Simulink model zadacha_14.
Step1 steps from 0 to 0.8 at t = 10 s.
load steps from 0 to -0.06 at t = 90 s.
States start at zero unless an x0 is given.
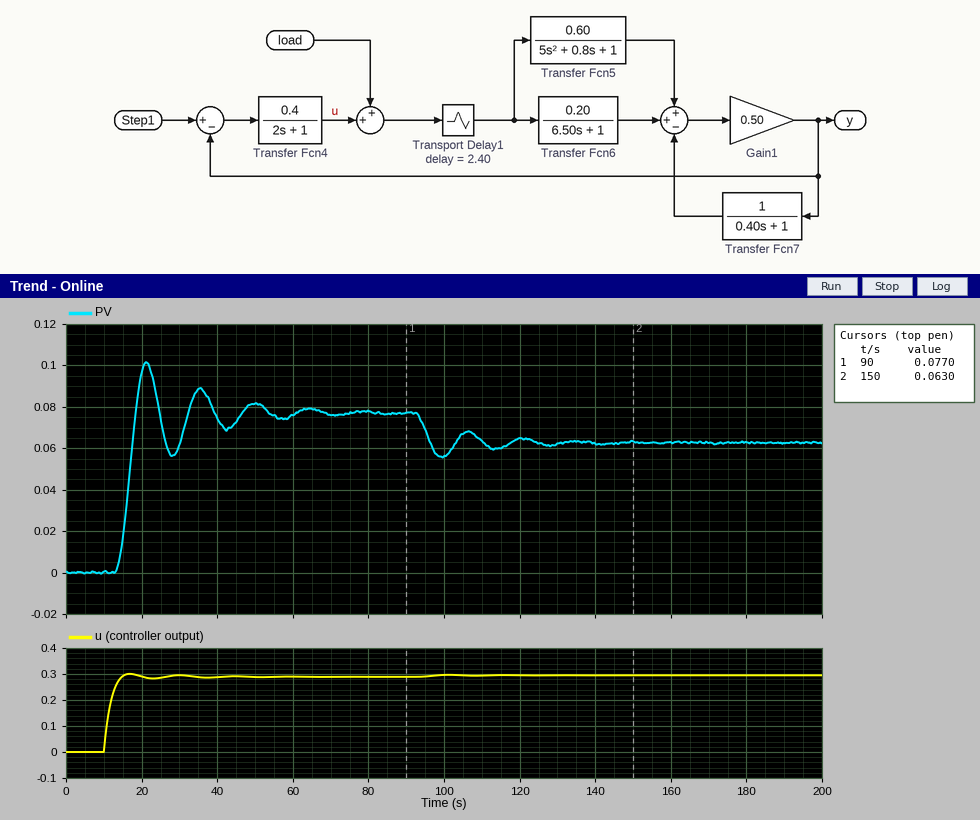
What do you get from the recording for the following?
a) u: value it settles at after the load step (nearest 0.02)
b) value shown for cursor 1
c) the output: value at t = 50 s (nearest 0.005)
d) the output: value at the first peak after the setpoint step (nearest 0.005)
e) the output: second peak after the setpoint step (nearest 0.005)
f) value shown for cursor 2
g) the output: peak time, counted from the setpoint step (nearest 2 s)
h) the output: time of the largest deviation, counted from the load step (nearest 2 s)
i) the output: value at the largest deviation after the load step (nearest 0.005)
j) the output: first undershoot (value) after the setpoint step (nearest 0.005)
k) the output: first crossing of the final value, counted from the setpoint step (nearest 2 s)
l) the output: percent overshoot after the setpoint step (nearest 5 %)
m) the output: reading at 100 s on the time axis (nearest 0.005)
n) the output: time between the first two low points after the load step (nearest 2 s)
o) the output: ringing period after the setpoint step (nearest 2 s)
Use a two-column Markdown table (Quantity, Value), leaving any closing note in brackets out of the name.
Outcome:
| Quantity | Value |
|---|---|
| u: value it settles at after the load step | 0.30 |
| value shown for cursor 1 | 0.0770 |
| the output: value at t = 50 s | 0.080 |
| the output: value at the first peak after the setpoint step | 0.100 |
| the output: second peak after the setpoint step | 0.090 |
| value shown for cursor 2 | 0.0630 |
| the output: peak time, counted from the setpoint step | 12 s |
| the output: time of the largest deviation, counted from the load step | 10 s |
| the output: value at the largest deviation after the load step | 0.055 |
| the output: first undershoot (value) after the setpoint step | 0.055 |
| the output: first crossing of the final value, counted from the setpoint step | 8 s |
| the output: percent overshoot after the setpoint step | 30 % |
| the output: reading at 100 s on the time axis | 0.055 |
| the output: time between the first two low points after the load step | 14 s |
| the output: ringing period after the setpoint step | 14 s |
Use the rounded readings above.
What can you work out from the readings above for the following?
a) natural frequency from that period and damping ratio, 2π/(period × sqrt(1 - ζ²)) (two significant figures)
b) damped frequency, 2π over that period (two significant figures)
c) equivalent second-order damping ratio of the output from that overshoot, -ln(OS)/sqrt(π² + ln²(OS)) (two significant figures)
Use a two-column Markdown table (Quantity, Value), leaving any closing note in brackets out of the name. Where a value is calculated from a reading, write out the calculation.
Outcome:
| Quantity | Value |
|---|---|
| natural frequency from that period and damping ratio, 2π/(period × sqrt(1 - ζ²)) | 2π / (14 × sqrt(1 - 0.36²)) = 0.48 rad/s |
| damped frequency, 2π over that period | 2π / 14 = 0.45 rad/s |
| equivalent second-order damping ratio of the output from that overshoot, -ln(OS)/sqrt(π² + ln²(OS)) | ln(0.3) = -1.204; 1.204 / sqrt(9.870 + 1.450) = 0.36 |
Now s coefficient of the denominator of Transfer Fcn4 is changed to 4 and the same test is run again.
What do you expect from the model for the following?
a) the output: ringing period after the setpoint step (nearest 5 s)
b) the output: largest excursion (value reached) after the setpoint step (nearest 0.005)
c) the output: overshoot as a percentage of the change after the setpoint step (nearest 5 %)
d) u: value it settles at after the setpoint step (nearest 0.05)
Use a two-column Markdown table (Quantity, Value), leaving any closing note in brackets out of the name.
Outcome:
| Quantity | Value |
|---|---|
| the output: ringing period after the setpoint step | 15 s |
| the output: largest excursion (value reached) after the setpoint step | 0.085 |
| the output: overshoot as a percentage of the change after the setpoint step | 10 % |
| u: value it settles at after the setpoint step | 0.30 |
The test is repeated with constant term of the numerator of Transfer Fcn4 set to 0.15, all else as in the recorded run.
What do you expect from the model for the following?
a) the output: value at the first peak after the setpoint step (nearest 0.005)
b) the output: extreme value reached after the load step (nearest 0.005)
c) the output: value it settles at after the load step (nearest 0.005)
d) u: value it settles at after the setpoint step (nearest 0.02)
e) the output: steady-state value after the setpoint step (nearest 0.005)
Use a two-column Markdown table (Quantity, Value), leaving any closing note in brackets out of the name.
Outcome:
| Quantity | Value |
|---|---|
| the output: value at the first peak after the setpoint step | 0.040 |
| the output: extreme value reached after the load step | 0.010 |
| the output: value it settles at after the load step | 0.015 |
| u: value it settles at after the setpoint step | 0.12 |
| the output: steady-state value after the setpoint step | 0.030 |
